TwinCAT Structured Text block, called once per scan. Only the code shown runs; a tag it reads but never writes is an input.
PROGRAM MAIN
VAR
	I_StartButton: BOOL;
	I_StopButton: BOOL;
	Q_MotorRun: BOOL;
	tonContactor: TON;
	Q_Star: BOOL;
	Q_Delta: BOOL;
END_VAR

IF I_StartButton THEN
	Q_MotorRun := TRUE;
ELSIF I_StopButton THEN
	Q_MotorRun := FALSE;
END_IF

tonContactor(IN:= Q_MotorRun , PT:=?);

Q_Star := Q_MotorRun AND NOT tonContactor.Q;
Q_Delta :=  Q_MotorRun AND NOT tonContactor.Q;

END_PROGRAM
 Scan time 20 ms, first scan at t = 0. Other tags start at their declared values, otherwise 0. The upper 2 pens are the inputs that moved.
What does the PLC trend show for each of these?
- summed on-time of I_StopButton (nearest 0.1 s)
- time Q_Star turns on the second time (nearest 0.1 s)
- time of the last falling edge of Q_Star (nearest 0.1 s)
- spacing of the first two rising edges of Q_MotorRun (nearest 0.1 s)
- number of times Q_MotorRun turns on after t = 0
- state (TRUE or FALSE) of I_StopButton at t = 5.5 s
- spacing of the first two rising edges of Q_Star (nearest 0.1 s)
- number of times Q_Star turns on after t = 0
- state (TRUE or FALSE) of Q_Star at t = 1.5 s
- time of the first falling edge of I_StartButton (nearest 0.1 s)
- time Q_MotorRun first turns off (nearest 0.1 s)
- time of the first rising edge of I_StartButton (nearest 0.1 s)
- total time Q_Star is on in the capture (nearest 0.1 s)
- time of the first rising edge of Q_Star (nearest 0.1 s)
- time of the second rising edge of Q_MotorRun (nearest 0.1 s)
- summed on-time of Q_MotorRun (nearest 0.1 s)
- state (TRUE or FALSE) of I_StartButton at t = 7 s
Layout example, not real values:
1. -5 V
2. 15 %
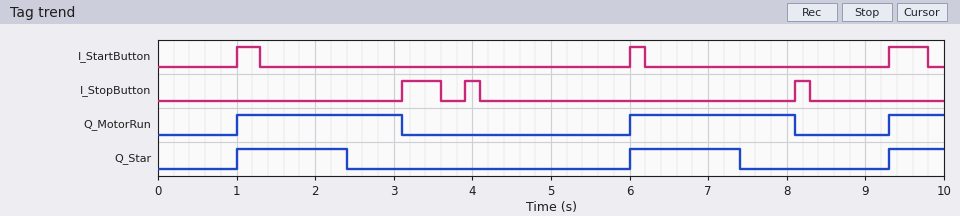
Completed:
1. 0.9 s
2. 6.0 s
3. 7.4 s
4. 5.0 s
5. 3
6. FALSE
7. 5.0 s
8. 3
9. TRUE
10. 1.3 s
11. 3.1 s
12. 1.0 s
13. 3.5 s
14. 1.0 s
15. 6.0 s
16. 4.9 s
17. FALSE
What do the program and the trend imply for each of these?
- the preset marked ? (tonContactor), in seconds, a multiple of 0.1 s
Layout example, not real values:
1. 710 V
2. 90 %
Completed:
1. 1.4 s
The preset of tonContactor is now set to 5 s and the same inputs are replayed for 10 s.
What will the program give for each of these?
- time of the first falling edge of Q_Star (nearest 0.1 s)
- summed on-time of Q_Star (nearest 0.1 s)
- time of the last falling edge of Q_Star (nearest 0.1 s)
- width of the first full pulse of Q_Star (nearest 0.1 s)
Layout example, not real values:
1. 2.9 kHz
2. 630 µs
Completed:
1. 3.1 s
2. 4.9 s
3. 8.1 s
4. 2.1 s
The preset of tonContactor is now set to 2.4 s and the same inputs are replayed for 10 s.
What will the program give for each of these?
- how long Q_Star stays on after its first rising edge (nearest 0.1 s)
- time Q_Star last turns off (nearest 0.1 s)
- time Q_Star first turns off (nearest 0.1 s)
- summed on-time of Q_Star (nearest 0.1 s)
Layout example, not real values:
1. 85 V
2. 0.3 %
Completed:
1. 2.1 s
2. 8.1 s
3. 3.1 s
4. 4.9 s
